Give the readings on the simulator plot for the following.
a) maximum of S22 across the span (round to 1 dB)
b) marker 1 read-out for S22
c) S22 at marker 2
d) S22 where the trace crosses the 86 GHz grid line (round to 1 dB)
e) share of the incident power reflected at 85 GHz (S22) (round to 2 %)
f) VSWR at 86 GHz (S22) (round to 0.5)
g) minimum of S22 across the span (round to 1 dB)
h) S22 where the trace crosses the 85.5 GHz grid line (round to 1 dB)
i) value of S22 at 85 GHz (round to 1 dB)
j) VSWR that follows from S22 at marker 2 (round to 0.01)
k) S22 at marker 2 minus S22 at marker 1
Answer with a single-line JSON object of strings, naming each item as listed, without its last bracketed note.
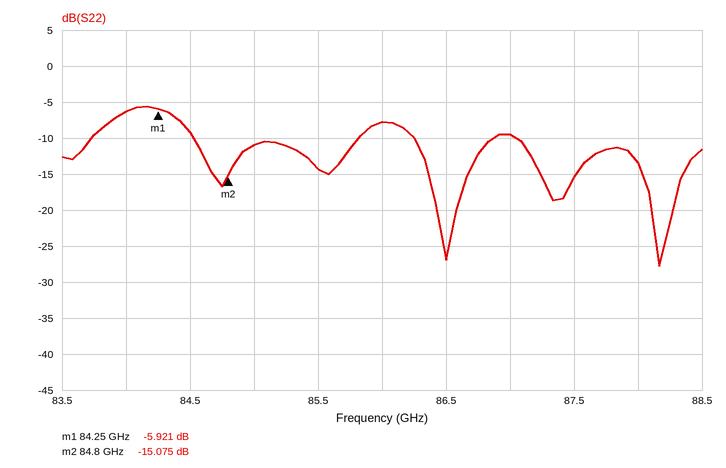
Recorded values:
{"maximum of S22 across the span": "-6 dB", "marker 1 read-out for S22": "-5.921 dB", "S22 at marker 2": "-15.075 dB", "S22 where the trace crosses the 86 GHz grid line": "-8 dB", "share of the incident power reflected at 85 GHz (S22)": "8 %", "VSWR at 86 GHz (S22)": "2.5", "minimum of S22 across the span": "-28 dB", "S22 where the trace crosses the 85.5 GHz grid line": "-14 dB", "value of S22 at 85 GHz": "-11 dB", "VSWR that follows from S22 at marker 2": "1.43", "S22 at marker 2 minus S22 at marker 1": "-9.154 dB"}
